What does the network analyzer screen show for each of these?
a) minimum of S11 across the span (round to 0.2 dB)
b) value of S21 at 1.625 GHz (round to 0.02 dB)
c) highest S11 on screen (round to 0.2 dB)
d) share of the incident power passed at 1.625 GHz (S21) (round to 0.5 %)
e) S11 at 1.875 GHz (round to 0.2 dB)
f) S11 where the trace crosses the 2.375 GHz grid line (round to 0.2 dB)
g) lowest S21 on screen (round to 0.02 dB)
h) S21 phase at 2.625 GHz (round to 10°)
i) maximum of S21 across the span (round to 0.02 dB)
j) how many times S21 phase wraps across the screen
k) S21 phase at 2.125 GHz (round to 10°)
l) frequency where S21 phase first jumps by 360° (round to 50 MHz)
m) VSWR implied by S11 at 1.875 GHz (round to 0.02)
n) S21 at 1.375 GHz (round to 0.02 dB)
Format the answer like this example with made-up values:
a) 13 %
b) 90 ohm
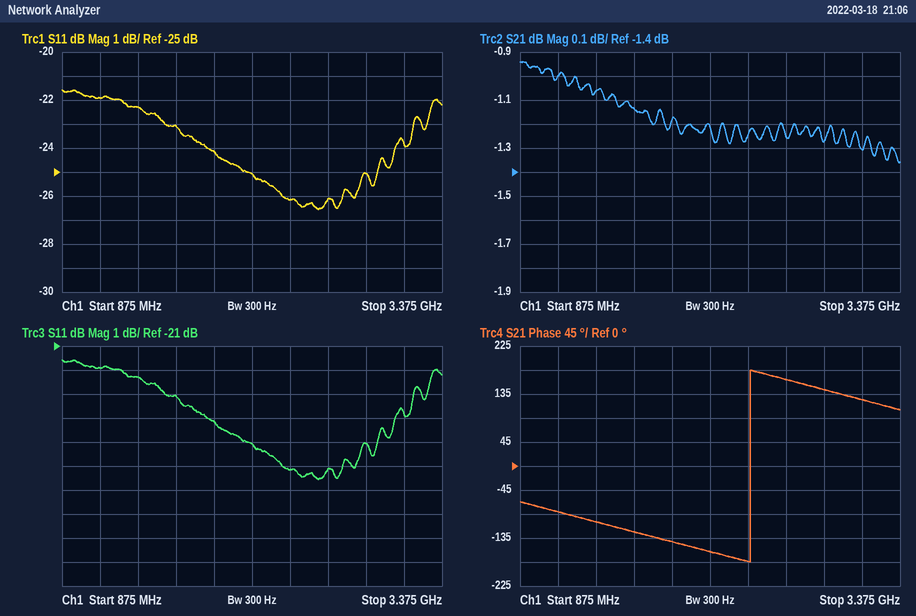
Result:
a) -26.6 dB
b) -1.14 dB
c) -21.6 dB
d) 77.0 %
e) -24.2 dB
f) -26.2 dB
g) -1.36 dB
h) 160°
i) -0.94 dB
j) 1
k) -160°
l) 2.40 GHz
m) 1.14
n) -1.06 dB
